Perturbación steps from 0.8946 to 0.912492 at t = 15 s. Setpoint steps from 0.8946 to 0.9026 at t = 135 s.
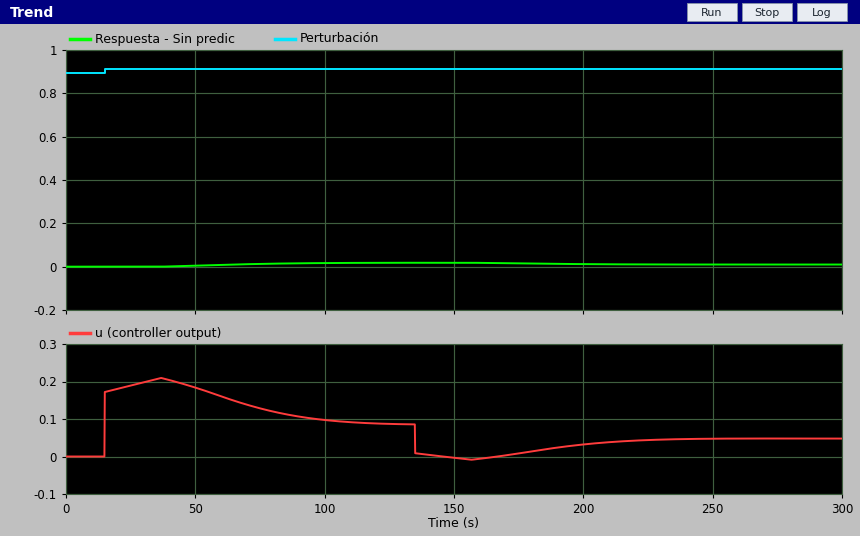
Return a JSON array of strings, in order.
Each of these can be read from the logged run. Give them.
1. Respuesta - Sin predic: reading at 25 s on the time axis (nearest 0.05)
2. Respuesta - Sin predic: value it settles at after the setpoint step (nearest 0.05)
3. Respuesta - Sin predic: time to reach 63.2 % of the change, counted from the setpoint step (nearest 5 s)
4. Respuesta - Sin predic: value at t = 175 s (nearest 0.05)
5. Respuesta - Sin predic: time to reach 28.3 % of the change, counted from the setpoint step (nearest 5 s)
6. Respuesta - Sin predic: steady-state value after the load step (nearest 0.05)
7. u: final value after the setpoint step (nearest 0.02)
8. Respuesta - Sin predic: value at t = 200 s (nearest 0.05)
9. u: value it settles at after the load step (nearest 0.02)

["0.00", "0.00", "55 s", "0.00", "35 s", "0.00", "0.08", "0.00", "0.04"]
